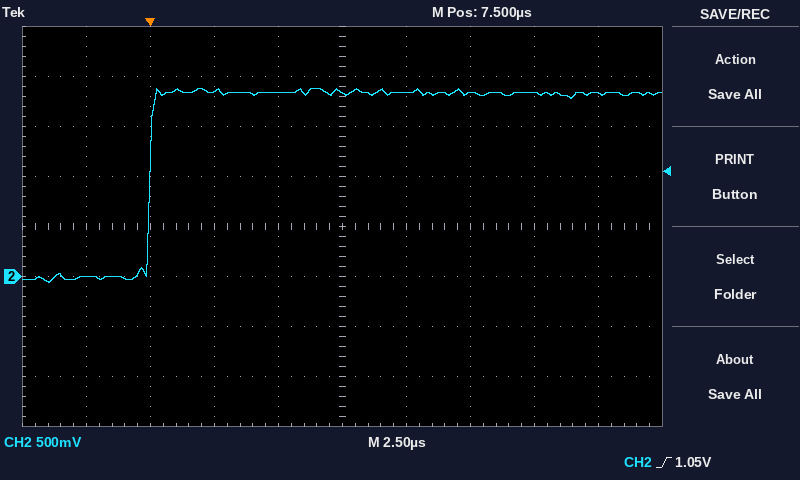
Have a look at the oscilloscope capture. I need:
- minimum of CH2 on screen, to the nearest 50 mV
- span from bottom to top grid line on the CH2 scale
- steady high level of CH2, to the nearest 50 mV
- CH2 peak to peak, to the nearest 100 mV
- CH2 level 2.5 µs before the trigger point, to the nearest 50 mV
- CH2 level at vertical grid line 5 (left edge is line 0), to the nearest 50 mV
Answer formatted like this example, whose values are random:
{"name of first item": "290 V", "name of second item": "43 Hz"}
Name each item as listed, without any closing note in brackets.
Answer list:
{"minimum of CH2 on screen, to the nearest 50 mV": "-50 mV", "span from bottom to top grid line on the CH2 scale": "4 V", "steady high level of CH2, to the nearest 50 mV": "1.85 V", "CH2 peak to peak, to the nearest 100 mV": "1.90 V", "CH2 level 2.5 µs before the trigger point, to the nearest 50 mV": "0 mV", "CH2 level at vertical grid line 5 (left edge is line 0), to the nearest 50 mV": "1.85 V"}
